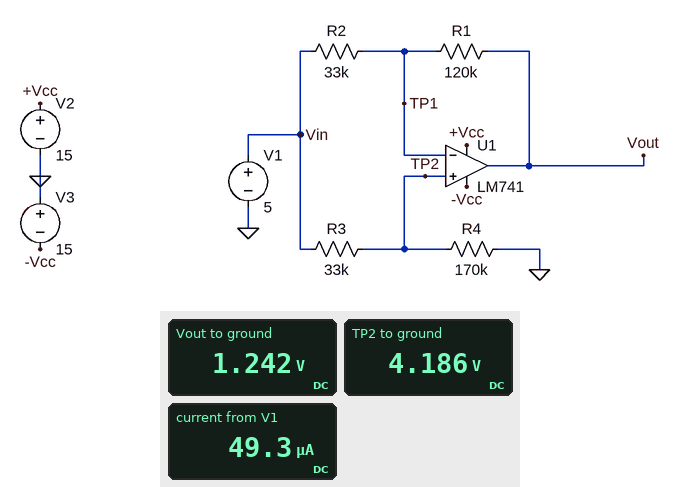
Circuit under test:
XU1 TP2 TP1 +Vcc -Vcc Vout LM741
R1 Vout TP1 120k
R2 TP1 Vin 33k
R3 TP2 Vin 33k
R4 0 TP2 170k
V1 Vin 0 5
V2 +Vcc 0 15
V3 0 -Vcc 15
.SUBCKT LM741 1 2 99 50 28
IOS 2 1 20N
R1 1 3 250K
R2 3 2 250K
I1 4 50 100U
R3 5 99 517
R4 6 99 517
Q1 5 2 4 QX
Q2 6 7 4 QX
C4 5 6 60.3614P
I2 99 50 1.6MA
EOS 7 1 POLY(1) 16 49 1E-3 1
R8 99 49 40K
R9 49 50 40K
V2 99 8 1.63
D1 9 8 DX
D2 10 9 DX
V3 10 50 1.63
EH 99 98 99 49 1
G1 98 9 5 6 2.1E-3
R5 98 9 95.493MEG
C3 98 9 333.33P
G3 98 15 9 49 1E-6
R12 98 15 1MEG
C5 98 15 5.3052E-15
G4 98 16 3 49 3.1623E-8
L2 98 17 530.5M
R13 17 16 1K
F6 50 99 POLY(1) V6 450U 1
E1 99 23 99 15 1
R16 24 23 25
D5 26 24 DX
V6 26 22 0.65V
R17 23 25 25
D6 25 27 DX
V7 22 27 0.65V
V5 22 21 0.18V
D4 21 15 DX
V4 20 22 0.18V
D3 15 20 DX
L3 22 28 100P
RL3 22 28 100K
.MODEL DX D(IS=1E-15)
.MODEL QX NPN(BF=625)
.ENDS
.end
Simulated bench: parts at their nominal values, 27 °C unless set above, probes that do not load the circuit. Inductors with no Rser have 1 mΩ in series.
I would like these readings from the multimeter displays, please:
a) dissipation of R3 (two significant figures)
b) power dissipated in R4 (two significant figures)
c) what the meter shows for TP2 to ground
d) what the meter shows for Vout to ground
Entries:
20 µW
100 µW
4.186 V
1.242 V
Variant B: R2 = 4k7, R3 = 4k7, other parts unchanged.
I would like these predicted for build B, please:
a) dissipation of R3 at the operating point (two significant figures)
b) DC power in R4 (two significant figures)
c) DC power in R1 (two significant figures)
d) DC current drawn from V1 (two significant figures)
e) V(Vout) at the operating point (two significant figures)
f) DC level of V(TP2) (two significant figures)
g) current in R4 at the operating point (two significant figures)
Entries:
3.9 µW
140 µW
96 µW
57 µA
1.5 V
4.9 V
29 µA
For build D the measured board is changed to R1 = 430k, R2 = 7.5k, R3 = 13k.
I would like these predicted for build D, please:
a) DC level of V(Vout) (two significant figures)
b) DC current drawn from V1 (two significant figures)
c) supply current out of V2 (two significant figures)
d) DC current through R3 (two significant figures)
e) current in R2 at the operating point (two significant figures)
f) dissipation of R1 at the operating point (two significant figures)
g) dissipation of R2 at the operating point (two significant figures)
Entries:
-14 V
71 µA
1.6 mA
27 µA
44 µA
810 µW
14 µW
